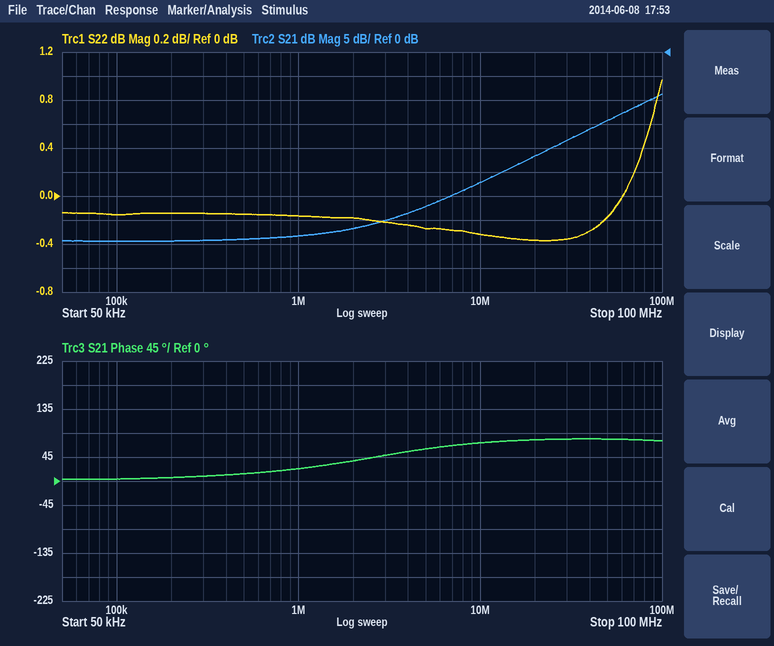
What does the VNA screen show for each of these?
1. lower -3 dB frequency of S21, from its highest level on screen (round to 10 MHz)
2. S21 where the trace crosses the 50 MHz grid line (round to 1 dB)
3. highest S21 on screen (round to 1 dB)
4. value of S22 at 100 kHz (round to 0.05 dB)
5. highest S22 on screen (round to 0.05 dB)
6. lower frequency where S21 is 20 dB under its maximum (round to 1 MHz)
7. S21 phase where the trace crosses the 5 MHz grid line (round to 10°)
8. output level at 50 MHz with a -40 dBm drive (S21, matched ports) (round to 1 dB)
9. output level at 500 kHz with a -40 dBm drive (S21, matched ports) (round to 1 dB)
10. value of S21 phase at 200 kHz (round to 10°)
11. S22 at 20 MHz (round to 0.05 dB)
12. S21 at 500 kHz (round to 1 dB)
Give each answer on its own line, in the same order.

70 MHz
-14 dB
-9 dB
-0.15 dB
0.95 dB
8 MHz
60°
-54 dBm
-79 dBm
10°
-0.35 dB
-39 dB
